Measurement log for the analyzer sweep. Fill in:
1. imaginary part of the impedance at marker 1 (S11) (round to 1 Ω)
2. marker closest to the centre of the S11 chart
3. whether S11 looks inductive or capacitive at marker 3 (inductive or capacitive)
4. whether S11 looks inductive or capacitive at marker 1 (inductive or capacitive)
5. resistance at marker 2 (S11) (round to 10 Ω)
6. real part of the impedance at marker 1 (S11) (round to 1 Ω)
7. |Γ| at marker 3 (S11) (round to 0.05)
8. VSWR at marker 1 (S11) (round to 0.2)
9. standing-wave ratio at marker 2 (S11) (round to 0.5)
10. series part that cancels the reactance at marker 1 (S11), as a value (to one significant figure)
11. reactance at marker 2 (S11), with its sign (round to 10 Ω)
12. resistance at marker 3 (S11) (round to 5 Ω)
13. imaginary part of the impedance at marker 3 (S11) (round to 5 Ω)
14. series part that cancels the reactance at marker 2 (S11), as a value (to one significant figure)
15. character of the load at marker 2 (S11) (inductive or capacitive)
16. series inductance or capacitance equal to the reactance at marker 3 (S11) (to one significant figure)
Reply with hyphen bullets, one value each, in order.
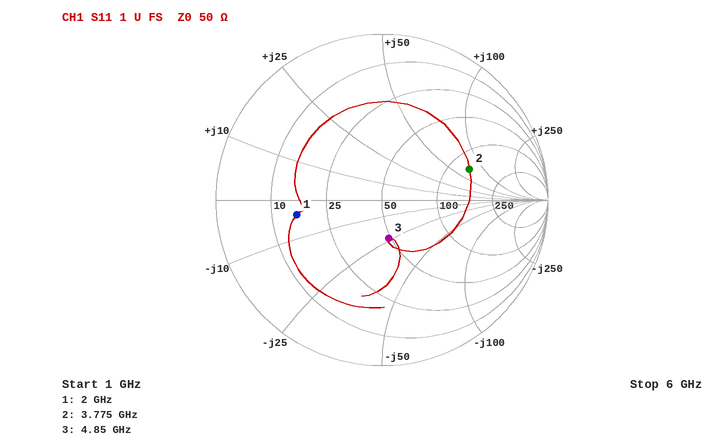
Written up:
- -4 Ω
- marker 3
- capacitive
- capacitive
- 130 Ω
- 16 Ω
- 0.25
- 3.2
- 3.5
- 300 pH
- +70 Ω
- 50 Ω
- -25 Ω
- 600 fF
- inductive
- 1 pF
